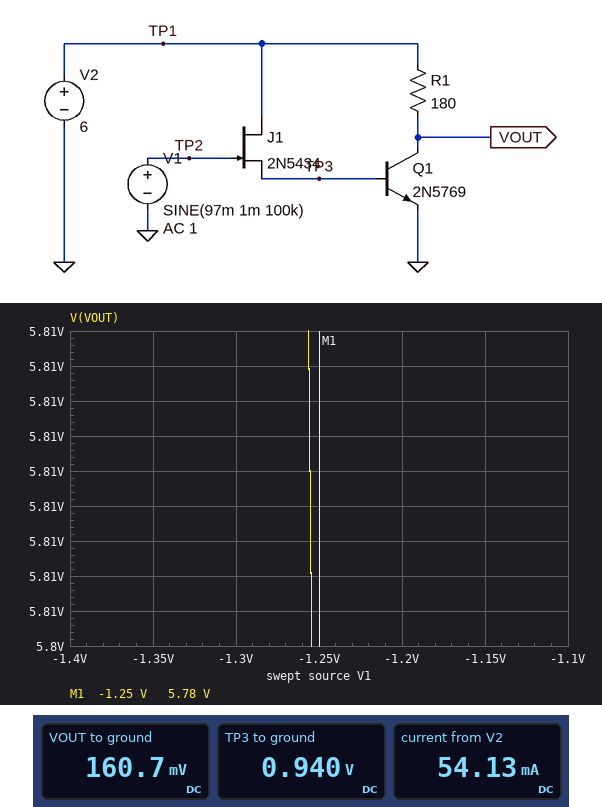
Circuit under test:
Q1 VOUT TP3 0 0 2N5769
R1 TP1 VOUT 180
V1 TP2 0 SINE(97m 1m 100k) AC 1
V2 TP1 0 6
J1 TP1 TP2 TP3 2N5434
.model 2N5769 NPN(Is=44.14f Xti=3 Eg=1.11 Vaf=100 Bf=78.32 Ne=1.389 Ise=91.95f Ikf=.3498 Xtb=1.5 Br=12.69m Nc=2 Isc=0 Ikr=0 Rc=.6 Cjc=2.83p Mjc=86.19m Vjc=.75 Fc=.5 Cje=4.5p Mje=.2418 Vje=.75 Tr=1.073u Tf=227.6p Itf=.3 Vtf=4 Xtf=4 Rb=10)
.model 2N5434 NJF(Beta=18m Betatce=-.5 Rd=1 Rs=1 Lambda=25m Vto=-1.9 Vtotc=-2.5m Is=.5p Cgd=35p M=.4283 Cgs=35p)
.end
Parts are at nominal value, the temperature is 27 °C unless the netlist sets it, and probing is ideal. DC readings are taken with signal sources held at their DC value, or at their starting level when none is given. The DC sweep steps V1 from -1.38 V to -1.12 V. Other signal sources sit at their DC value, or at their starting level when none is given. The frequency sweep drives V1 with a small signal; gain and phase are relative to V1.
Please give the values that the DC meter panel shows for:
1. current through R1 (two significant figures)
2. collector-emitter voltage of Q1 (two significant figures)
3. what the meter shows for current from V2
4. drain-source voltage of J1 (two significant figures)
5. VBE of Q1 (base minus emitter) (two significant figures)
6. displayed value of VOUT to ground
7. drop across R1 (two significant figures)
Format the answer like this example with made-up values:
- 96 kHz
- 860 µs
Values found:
- 32 mA
- 160 mV
- 54.13 mA
- 5.1 V
- 940 mV
- 160.7 mV
- 5.8 V
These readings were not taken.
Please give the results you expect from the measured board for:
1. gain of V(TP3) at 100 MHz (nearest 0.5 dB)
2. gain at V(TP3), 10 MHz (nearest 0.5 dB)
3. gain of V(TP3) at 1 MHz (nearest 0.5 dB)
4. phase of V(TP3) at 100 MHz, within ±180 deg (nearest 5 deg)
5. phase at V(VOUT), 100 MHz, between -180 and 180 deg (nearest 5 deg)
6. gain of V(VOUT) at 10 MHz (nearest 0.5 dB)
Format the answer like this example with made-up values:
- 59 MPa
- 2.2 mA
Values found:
- -10.0 dB
- -10.5 dB
- -10.5 dB
- 15 deg
- 20 deg
- -35.0 dB
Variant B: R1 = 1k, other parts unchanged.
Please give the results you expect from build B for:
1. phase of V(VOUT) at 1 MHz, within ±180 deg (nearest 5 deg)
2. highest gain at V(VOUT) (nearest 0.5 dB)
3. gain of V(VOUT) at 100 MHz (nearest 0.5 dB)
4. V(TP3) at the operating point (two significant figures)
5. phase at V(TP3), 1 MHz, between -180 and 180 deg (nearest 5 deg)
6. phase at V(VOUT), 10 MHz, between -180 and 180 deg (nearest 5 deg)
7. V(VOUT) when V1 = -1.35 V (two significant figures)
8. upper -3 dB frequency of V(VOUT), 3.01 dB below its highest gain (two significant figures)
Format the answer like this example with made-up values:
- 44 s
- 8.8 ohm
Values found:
- 150 deg
- -28.0 dB
- -31.0 dB
- 930 mV
- 0 deg
- 60 deg
- 5.9 V
- 1.7 GHz
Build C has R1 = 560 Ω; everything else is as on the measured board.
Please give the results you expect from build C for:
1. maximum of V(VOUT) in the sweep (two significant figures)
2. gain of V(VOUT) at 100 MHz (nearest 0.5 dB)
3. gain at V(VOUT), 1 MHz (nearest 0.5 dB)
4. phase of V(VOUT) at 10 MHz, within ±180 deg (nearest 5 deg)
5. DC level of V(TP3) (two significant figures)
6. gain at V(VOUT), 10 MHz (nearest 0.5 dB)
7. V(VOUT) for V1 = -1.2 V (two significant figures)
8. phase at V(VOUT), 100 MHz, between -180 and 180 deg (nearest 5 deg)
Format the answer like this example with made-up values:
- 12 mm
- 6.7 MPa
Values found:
- 6.0 V
- -32.0 dB
- -41.0 dB
- 75 deg
- 930 mV
- -35.5 dB
- 4.0 V
- 15 deg
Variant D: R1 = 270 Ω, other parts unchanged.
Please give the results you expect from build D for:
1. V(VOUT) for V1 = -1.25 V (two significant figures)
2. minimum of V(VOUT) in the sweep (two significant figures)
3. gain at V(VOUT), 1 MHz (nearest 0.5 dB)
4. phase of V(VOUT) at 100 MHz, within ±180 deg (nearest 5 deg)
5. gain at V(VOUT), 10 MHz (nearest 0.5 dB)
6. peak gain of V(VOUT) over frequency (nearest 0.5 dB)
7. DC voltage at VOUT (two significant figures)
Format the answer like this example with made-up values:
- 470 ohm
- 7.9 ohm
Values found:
- 5.7 V
- 2.5 V
- -36.5 dB
- 15 deg
- -35.5 dB
- -32.0 dB
- 150 mV
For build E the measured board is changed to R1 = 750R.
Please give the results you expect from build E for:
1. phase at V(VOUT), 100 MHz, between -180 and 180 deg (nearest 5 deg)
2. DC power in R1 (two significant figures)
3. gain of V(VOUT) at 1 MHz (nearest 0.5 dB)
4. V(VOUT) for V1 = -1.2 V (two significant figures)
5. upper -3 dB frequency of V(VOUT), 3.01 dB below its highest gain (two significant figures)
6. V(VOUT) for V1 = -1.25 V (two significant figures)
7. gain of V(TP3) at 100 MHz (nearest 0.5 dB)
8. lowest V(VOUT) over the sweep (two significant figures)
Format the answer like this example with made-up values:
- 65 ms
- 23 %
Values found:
- 15 deg
- 46 mW
- -43.0 dB
- 3.3 V
- 1.6 GHz
- 5.1 V
- -10.0 dB
- 230 mV
